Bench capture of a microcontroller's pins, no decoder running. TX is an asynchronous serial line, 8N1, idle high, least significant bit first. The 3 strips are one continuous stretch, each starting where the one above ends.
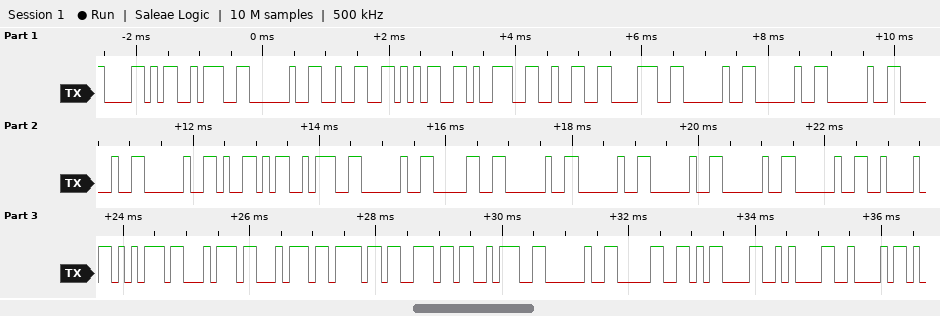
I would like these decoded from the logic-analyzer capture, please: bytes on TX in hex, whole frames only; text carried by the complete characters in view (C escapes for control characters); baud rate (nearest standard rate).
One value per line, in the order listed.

58 3A 20 32 35 39 32 38 20 20 20 20 20 59 3A 20 30 20 20 20 20 20 42 75 74 74 6F 6E 3A 20 30 0D 0A 42
"X: 25928     Y: 0     Button: 0\r\nB"
9600 baud
